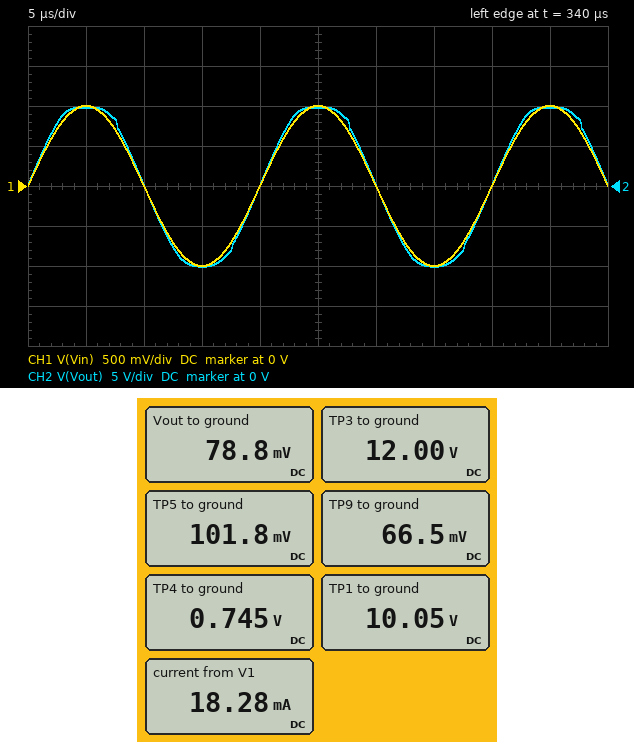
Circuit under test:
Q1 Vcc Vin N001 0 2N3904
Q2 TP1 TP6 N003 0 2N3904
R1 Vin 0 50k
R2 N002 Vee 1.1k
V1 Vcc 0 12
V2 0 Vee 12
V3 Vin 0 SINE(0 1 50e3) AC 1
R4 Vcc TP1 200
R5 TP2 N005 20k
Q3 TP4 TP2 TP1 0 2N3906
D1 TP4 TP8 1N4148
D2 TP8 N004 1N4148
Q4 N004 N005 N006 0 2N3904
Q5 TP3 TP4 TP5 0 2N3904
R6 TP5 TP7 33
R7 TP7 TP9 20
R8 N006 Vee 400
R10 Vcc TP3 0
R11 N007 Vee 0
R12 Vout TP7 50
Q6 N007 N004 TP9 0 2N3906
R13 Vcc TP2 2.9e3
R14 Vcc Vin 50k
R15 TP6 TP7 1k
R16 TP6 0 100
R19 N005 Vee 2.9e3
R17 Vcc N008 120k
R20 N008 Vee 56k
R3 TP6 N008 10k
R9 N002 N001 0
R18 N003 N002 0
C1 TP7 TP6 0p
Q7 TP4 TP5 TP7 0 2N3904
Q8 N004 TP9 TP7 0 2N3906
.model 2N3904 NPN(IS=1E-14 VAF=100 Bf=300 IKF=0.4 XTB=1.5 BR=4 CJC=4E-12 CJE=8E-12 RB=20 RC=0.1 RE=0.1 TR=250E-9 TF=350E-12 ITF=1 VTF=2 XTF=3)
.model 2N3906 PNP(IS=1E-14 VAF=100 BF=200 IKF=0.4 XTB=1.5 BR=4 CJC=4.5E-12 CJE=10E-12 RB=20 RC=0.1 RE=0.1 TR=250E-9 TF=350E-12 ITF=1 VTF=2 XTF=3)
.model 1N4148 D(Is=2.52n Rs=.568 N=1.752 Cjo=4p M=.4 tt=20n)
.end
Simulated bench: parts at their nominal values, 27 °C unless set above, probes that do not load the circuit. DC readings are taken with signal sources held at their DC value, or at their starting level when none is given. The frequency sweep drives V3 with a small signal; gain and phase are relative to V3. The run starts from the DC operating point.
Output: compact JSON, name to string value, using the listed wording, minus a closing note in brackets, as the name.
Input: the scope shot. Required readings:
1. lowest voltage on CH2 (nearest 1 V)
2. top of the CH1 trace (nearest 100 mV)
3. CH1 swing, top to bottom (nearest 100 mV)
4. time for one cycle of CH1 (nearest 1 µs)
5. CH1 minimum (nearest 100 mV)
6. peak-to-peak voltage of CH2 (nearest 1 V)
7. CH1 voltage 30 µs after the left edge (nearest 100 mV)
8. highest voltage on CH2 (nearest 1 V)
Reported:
{"lowest voltage on CH2": "-10 V", "top of the CH1 trace": "1.0 V", "CH1 swing, top to bottom": "2.0 V", "time for one cycle of CH1": "20 µs", "CH1 minimum": "-1.0 V", "peak-to-peak voltage of CH2": "20 V", "CH1 voltage 30 µs after the left edge": "0 V", "highest voltage on CH2": "10 V"}
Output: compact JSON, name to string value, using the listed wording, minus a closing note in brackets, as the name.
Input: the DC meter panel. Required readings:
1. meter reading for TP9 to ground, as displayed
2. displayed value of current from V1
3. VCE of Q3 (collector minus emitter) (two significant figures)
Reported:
{"meter reading for TP9 to ground, as displayed": "66.5 mV", "displayed value of current from V1": "18.28 mA", "VCE of Q3 (collector minus emitter)": "-9.3 V"}
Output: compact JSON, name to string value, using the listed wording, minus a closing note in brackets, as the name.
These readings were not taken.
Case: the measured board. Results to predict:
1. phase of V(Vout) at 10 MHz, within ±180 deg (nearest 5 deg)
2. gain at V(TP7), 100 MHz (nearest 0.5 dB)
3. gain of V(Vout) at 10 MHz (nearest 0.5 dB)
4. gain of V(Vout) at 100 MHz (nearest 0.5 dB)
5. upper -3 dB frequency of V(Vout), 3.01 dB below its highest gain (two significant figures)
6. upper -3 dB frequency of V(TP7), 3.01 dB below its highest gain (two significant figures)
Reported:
{"phase of V(Vout) at 10 MHz, within ±180 deg": "-25 deg", "gain at V(TP7), 100 MHz": "3.0 dB", "gain of V(Vout) at 10 MHz": "21.0 dB", "gain of V(Vout) at 100 MHz": "3.0 dB", "upper -3 dB frequency of V(Vout), 3.01 dB below its highest gain": "28 MHz", "upper -3 dB frequency of V(TP7), 3.01 dB below its highest gain": "28 MHz"}
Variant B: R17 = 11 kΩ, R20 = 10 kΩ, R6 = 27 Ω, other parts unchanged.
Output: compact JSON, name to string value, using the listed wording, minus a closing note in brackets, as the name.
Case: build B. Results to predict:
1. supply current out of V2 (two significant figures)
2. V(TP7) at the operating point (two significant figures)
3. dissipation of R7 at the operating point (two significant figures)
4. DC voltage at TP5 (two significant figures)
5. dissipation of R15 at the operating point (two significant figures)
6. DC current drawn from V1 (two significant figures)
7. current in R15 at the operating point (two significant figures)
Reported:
{"supply current out of V2": "18 mA", "V(TP7) at the operating point": "26 mV", "dissipation of R7 at the operating point": "9.1 µW", "DC voltage at TP5": "45 mV", "dissipation of R15 at the operating point": "790 nW", "DC current drawn from V1": "20 mA", "current in R15 at the operating point": "28 µA"}
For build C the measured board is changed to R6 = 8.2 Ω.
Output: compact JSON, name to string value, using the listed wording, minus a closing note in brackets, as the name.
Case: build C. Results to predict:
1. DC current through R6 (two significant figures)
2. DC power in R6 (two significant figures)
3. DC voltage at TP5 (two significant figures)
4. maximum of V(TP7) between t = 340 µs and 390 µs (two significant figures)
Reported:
{"DC current through R6": "870 µA", "DC power in R6": "6.2 µW", "DC voltage at TP5": "86 mV", "maximum of V(TP7) between t = 340 µs and 390 µs": "10 V"}
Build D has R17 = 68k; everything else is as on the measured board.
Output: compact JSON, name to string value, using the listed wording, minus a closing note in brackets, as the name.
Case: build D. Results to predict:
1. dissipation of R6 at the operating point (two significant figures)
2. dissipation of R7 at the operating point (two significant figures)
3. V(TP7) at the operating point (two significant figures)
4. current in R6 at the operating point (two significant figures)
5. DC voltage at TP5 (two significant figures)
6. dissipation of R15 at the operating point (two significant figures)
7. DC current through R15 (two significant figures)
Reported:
{"dissipation of R6 at the operating point": "15 µW", "dissipation of R7 at the operating point": "8.4 µW", "V(TP7) at the operating point": "17 mV", "current in R6 at the operating point": "670 µA", "DC voltage at TP5": "39 mV", "dissipation of R15 at the operating point": "370 nW", "DC current through R15": "19 µA"}
